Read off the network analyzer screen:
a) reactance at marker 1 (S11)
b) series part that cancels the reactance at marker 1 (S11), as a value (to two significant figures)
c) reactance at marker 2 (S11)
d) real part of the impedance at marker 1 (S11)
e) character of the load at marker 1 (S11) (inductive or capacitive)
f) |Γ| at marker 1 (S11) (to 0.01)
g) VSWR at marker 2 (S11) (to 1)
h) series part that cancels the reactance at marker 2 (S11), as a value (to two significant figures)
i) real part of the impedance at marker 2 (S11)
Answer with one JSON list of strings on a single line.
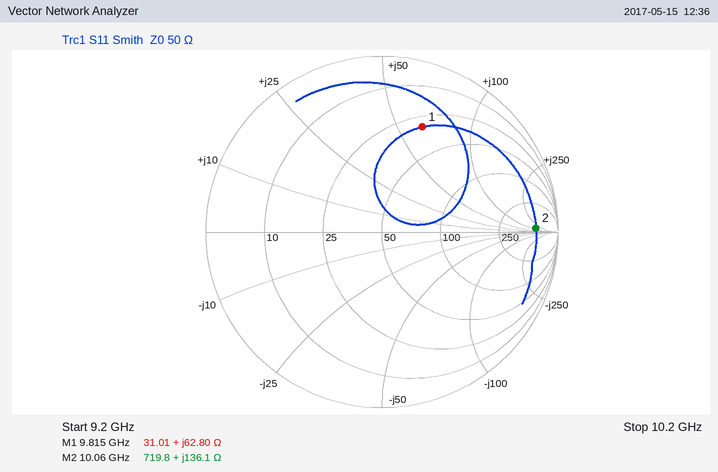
["+62.80 Ω", "260 fF", "+136.1 Ω", "31.01 Ω", "inductive", "0.64", "15", "120 fF", "719.8 Ω"]
